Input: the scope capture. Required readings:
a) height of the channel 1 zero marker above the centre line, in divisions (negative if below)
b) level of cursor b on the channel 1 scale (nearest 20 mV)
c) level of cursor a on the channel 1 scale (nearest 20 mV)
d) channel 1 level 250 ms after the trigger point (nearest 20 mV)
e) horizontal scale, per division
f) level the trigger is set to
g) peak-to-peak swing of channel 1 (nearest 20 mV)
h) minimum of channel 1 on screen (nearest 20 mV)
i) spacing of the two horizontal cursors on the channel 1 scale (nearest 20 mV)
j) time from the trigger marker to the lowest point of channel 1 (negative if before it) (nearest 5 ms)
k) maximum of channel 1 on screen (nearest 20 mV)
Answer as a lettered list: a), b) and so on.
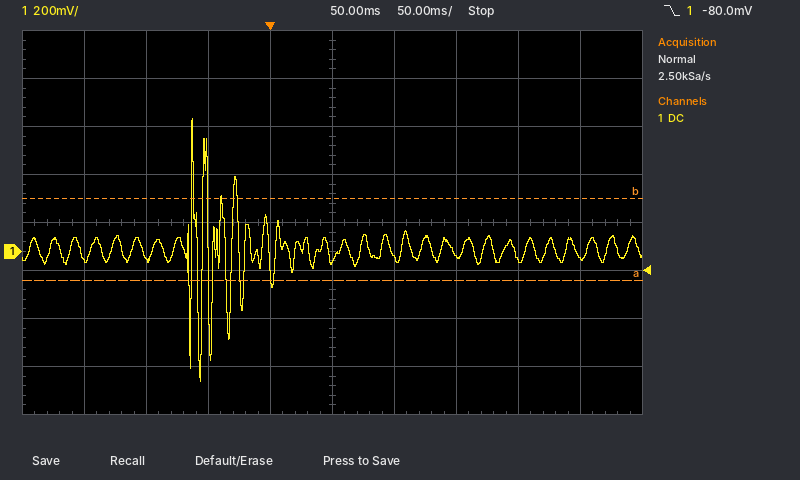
a) -0.6 div
b) 220 mV
c) -120 mV
d) -20 mV
e) 50 ms
f) -80.0 mV
g) 1.10 V
h) -540 mV
i) 340 mV
j) -55 ms
k) 560 mV
